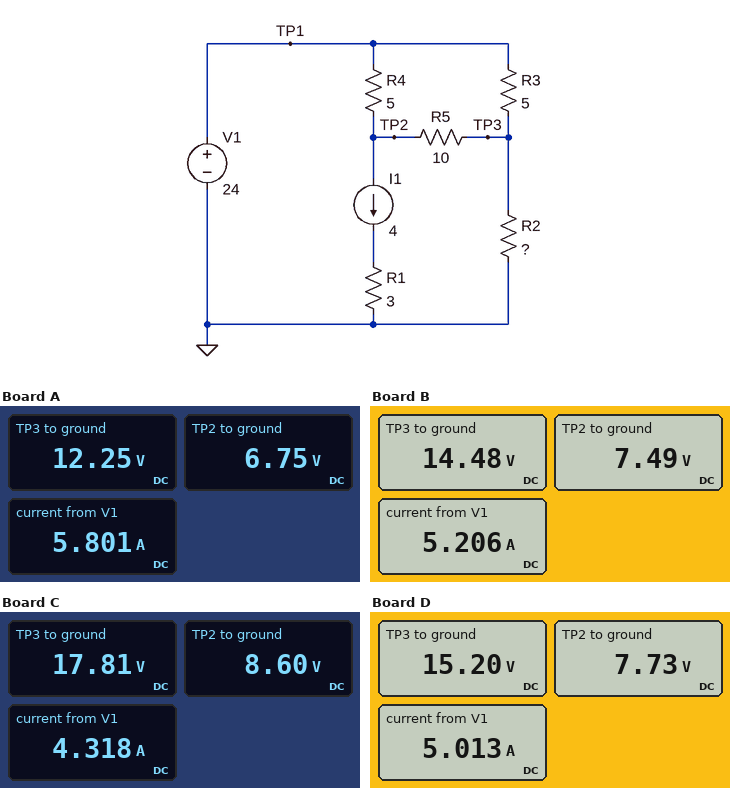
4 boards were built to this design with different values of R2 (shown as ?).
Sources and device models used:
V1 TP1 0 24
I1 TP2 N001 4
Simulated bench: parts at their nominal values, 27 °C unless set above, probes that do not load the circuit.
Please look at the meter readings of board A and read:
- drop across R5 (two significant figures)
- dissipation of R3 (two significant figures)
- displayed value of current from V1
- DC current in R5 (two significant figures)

5.5 V
28 W
5.801 A
550 mA
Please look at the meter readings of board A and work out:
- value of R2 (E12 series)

6.8 Ω
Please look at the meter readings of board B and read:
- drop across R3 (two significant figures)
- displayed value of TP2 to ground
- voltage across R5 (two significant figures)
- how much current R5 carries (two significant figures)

9.5 V
7.49 V
7.0 V
700 mA
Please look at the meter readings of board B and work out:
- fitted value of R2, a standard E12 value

12 Ω
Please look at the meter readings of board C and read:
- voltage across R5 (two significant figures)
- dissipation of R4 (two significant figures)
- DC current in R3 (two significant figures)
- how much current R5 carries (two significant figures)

9.2 V
47 W
1.2 A
920 mA
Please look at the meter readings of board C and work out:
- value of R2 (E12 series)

56 Ω
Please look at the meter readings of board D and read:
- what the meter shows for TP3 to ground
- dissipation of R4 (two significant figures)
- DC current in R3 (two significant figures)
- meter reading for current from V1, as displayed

15.20 V
53 W
1.8 A
5.013 A
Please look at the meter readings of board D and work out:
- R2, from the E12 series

15 Ω
